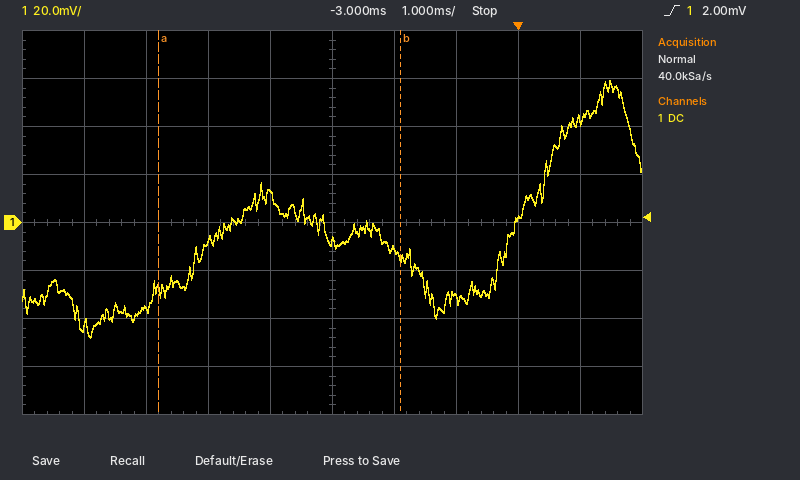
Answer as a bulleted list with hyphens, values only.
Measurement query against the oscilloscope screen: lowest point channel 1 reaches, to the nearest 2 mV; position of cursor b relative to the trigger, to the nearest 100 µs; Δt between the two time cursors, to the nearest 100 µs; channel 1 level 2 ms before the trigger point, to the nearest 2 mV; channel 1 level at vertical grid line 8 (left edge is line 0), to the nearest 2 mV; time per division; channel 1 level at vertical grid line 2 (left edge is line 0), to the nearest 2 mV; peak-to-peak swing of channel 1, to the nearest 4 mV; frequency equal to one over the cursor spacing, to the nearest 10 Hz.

- -48 mV
- -1.9 ms
- 3.9 ms
- -12 mV
- 2 mV
- 1 ms
- -36 mV
- 108 mV
- 260 Hz
